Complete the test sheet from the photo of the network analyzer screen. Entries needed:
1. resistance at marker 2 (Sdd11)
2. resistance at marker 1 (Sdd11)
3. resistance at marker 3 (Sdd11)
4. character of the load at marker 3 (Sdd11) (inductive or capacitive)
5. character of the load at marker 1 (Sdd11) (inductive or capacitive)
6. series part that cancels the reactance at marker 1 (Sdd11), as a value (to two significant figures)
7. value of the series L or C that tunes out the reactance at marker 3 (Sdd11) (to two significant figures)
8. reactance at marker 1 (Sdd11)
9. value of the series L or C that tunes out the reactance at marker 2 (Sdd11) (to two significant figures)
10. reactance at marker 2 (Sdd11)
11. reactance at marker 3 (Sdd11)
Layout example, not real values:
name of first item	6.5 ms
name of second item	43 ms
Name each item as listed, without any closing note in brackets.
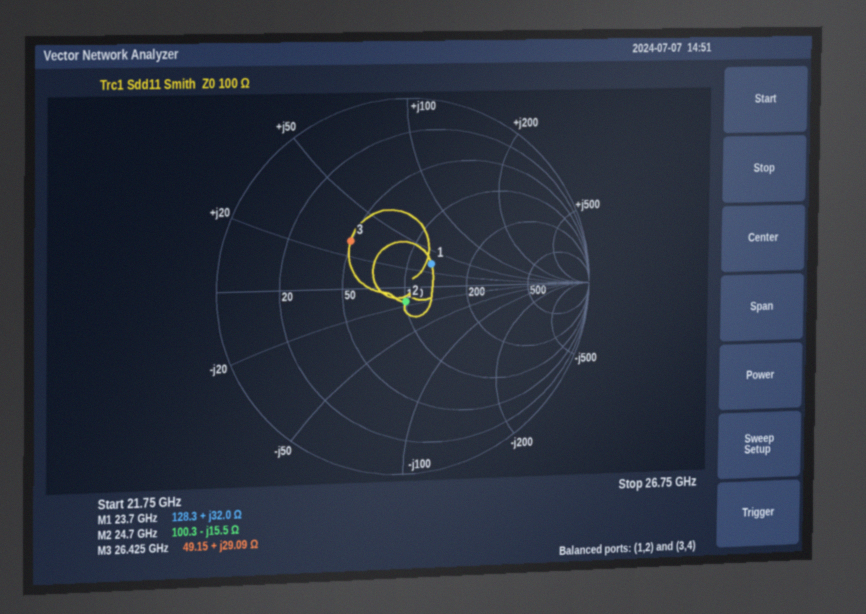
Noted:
resistance at marker 2	100.3 Ω
resistance at marker 1	128.3 Ω
resistance at marker 3	49.15 Ω
character of the load at marker 3 (Sdd11)	inductive
character of the load at marker 1 (Sdd11)	inductive
series part that cancels the reactance at marker 1 (Sdd11), as a value	210 fF
value of the series L or C that tunes out the reactance at marker 3 (Sdd11)	210 fF
reactance at marker 1	+32.0 Ω
value of the series L or C that tunes out the reactance at marker 2 (Sdd11)	100 pH
reactance at marker 2	-15.5 Ω
reactance at marker 3	+29.09 Ω
